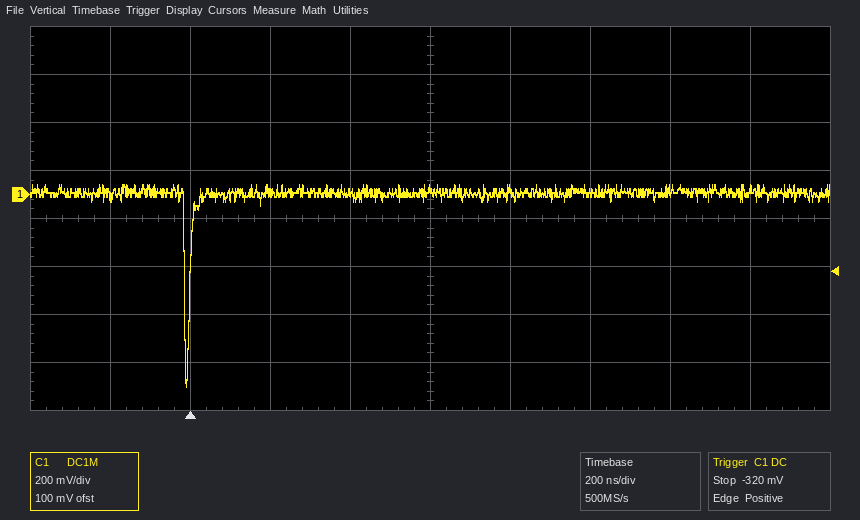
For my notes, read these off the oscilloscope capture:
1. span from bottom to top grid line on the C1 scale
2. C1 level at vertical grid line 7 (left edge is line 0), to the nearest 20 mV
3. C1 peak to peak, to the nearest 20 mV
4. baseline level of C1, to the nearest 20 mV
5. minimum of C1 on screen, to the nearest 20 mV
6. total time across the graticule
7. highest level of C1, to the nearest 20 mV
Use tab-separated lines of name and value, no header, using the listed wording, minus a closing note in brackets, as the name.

span from bottom to top grid line on the C1 scale	1.6 V
C1 level at vertical grid line 7 (left edge is line 0), to the nearest 20 mV	0 mV
C1 peak to peak, to the nearest 20 mV	840 mV
baseline level of C1, to the nearest 20 mV	0 mV
minimum of C1 on screen, to the nearest 20 mV	-800 mV
total time across the graticule	2 µs
highest level of C1, to the nearest 20 mV	40 mV
